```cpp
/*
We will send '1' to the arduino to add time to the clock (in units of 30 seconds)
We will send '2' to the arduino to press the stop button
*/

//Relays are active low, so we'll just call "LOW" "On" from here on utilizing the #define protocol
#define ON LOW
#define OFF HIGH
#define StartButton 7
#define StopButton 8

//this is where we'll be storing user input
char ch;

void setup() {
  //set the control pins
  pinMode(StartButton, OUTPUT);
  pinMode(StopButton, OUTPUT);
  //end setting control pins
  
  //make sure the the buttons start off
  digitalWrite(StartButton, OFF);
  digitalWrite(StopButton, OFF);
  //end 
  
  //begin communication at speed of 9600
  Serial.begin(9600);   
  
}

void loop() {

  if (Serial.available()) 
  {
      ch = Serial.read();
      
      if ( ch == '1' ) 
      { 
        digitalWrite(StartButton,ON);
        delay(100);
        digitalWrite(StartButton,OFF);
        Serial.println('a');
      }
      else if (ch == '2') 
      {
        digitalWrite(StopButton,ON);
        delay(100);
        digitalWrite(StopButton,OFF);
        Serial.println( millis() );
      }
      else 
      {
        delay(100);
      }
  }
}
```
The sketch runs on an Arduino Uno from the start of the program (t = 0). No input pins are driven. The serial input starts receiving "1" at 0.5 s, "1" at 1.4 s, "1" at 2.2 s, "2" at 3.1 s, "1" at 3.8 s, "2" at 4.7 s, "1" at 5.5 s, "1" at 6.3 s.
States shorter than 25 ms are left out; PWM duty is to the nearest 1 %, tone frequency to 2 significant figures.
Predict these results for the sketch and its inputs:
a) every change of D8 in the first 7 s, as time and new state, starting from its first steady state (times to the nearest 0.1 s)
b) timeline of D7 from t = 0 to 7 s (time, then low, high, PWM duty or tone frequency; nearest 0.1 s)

0 s high; 3.1 s low; 3.2 s high; 4.7 s low; 4.8 s high
0 s high; 0.5 s low; 0.6 s high; 1.4 s low; 1.5 s high; 2.2 s low; 2.3 s high; 3.8 s low; 3.9 s high; 5.5 s low; 5.6 s high; 6.3 s low; 6.4 s high
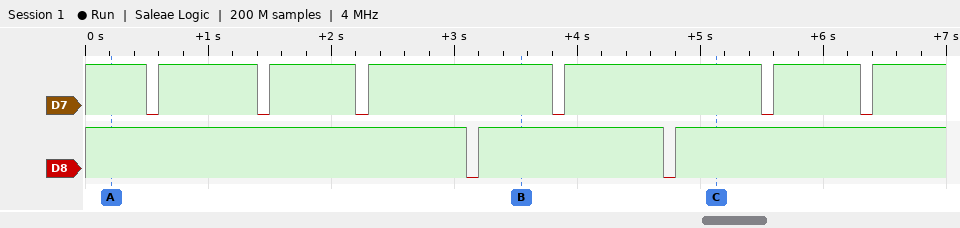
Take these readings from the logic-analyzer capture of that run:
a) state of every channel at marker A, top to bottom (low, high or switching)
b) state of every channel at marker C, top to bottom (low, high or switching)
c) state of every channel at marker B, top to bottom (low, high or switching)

D7 high, D8 high
D7 high, D8 high
D7 high, D8 high
